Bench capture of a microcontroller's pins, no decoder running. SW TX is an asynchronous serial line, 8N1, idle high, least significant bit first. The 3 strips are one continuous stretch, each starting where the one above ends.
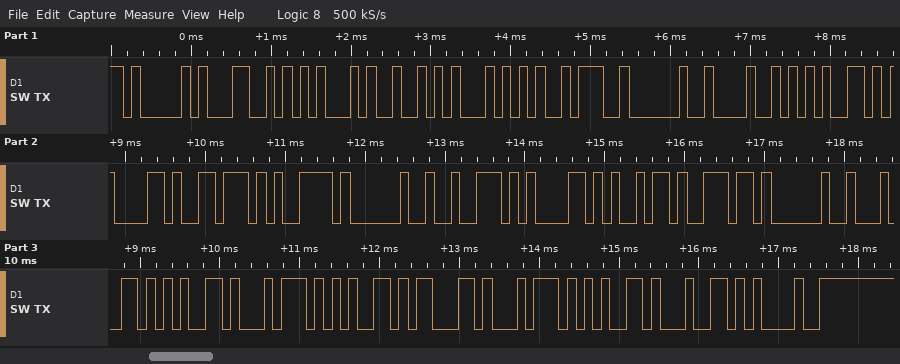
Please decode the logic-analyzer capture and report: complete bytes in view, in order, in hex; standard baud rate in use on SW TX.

41 4C 45 52 54 3A 20 48 65 61 76 79 20 72 61 69 6E 20 64 65 74 65 63 74 65 64 21
9600 baud
